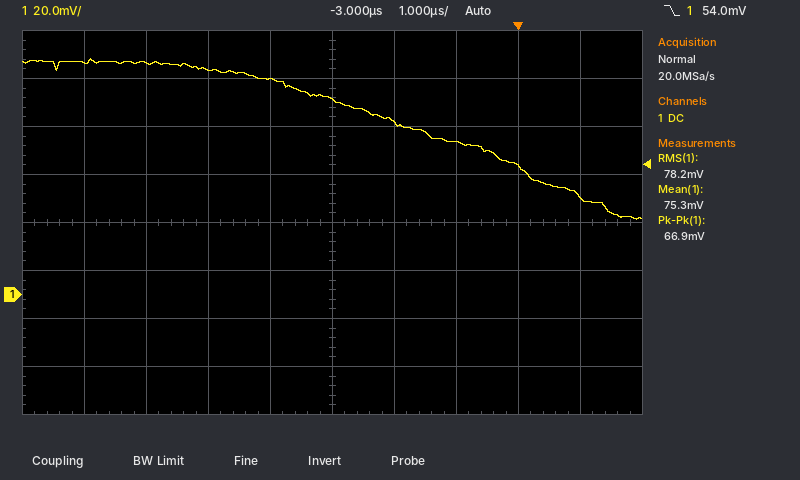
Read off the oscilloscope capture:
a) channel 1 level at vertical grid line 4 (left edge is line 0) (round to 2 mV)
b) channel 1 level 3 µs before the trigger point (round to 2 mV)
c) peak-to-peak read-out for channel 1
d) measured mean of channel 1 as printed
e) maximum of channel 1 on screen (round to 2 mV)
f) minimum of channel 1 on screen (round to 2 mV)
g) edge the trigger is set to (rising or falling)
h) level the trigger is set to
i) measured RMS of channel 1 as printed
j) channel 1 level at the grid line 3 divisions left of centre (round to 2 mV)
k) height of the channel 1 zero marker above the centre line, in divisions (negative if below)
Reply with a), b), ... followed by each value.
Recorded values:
a) 90 mV
b) 82 mV
c) 66.9 mV
d) 75.3 mV
e) 98 mV
f) 32 mV
g) falling
h) 54.0 mV
i) 78.2 mV
j) 96 mV
k) -1.5 div
